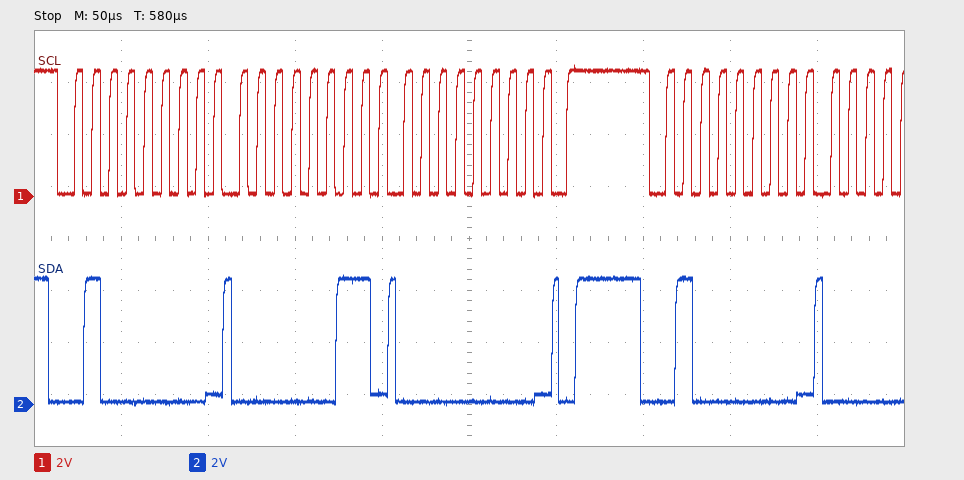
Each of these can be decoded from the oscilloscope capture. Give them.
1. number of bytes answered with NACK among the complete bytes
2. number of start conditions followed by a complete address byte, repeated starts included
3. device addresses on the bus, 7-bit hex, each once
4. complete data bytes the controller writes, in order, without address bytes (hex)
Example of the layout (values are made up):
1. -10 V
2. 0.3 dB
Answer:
1. 0
2. 2
3. 0x20
4. 03 00
